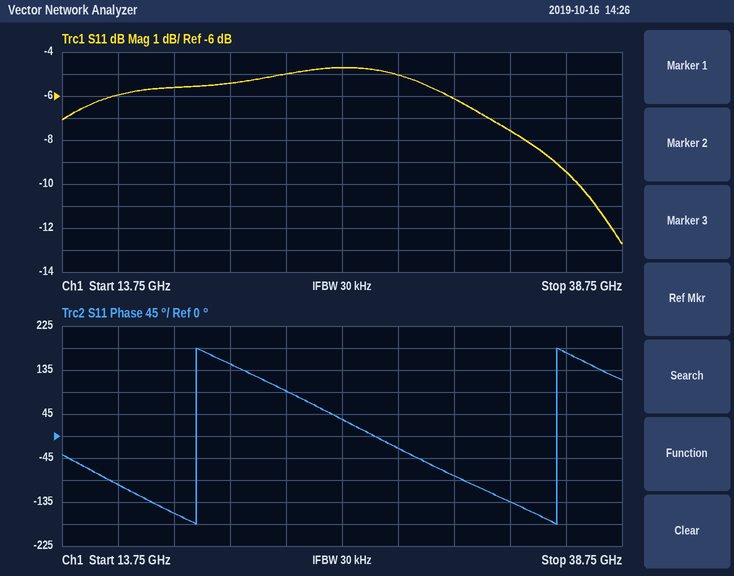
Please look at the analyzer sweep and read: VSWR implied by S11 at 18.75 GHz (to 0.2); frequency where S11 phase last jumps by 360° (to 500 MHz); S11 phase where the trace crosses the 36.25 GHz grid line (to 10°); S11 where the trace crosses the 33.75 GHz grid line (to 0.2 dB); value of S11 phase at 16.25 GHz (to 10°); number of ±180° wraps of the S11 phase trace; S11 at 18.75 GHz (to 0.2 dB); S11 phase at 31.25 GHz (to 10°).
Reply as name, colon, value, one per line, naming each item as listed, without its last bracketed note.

VSWR implied by S11 at 18.75 GHz: 3.2
frequency where S11 phase last jumps by 360°: 36.0 GHz
S11 phase where the trace crosses the 36.25 GHz grid line: 170°
S11 where the trace crosses the 33.75 GHz grid line: -7.6 dB
value of S11 phase at 16.25 GHz: -100°
number of ±180° wraps of the S11 phase trace: 2
S11 at 18.75 GHz: -5.6 dB
S11 phase at 31.25 GHz: -80°
